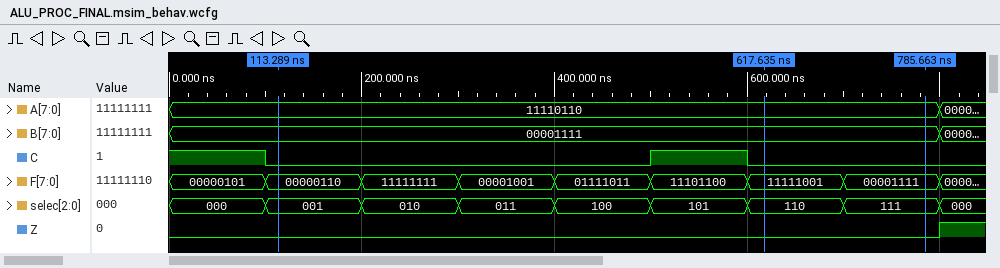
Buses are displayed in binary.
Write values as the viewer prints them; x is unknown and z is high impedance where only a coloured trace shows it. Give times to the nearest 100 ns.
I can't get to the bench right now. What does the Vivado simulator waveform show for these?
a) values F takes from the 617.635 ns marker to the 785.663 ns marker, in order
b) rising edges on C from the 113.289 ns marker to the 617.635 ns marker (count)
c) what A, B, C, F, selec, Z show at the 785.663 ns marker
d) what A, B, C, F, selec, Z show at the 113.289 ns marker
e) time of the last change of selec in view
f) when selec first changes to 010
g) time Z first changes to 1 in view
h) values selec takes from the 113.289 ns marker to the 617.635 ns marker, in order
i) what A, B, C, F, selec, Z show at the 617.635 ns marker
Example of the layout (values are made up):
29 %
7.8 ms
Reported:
11111001, 00001111
1
A=11110110, B=00001111, C=0, F=00001111, selec=111, Z=0
A=11110110, B=00001111, C=0, F=00000110, selec=001, Z=0
800 ns
200 ns
800 ns
001, 010, 011, 100, 101, 110
A=11110110, B=00001111, C=0, F=11111001, selec=110, Z=0
